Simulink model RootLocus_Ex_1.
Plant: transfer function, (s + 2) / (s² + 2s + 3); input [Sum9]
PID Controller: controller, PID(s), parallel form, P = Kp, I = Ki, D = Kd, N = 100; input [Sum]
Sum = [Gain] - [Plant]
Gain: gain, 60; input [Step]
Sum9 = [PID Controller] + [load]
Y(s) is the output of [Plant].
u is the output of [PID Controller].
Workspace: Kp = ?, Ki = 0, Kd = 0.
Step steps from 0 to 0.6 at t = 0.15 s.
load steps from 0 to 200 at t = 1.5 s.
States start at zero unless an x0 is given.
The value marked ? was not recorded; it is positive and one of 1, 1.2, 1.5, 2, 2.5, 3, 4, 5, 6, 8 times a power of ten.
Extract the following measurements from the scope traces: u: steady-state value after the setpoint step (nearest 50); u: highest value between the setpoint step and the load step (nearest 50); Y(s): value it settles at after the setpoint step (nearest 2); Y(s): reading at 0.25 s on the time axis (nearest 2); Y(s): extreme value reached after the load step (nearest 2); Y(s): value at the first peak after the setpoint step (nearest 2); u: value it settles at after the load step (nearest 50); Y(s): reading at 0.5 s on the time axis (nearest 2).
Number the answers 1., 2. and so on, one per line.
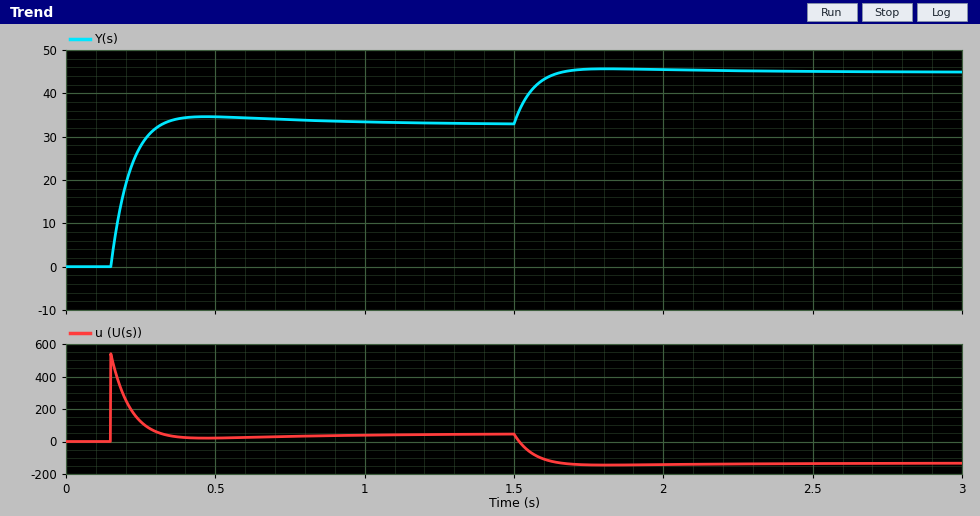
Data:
1. 50
2. 550
3. 32
4. 28
5. 46
6. 34
7. -150
8. 34
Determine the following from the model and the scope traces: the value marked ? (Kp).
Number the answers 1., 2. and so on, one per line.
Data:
1. 15
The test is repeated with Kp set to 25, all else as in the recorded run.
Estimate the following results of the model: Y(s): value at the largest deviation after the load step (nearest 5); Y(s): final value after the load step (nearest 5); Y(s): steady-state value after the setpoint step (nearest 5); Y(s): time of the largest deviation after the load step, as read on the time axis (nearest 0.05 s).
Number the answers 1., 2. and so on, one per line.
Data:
1. 40
2. 40
3. 35
4. 1.70 s
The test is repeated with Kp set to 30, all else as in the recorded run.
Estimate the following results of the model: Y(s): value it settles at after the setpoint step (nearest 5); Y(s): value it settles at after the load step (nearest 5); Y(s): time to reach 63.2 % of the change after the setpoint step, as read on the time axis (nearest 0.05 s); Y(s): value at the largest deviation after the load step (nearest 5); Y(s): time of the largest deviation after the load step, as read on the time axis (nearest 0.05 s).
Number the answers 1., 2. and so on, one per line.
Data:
1. 35
2. 40
3. 0.20 s
4. 40
5. 1.70 s
